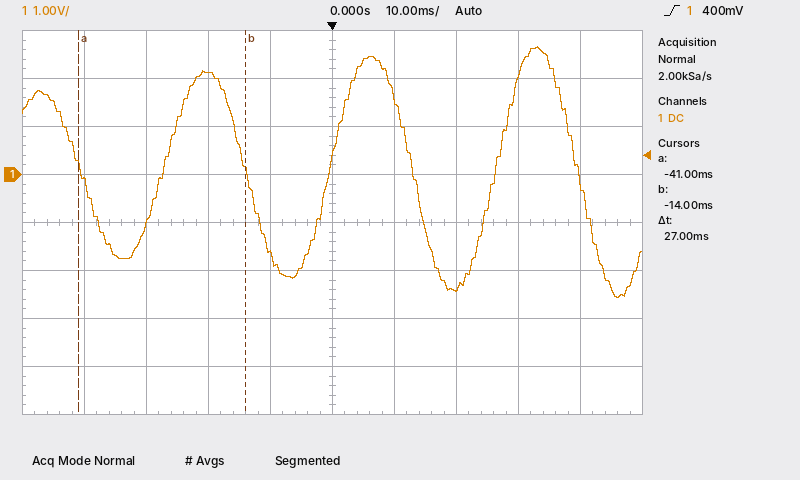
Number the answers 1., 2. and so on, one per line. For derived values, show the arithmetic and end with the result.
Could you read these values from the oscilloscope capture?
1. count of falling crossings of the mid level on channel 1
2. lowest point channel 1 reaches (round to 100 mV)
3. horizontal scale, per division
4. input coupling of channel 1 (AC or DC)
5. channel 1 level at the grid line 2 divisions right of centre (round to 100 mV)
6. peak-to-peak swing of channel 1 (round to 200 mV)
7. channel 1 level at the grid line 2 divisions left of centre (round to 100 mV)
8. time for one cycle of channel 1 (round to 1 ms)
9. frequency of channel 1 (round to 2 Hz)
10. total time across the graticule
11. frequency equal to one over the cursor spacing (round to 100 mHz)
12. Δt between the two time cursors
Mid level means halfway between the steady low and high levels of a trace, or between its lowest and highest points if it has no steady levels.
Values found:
1. 4
2. -2.6 V
3. 10 ms
4. DC
5. -2.4 V
6. 5.2 V
7. 2.1 V
8. 27 ms
9. 1 / 27 ms ≈ 37.0 Hz, so 38 Hz to the nearest 2 Hz
10. 100 ms
11. 1 / 27 ms ≈ 37.0 Hz
12. 27 ms
